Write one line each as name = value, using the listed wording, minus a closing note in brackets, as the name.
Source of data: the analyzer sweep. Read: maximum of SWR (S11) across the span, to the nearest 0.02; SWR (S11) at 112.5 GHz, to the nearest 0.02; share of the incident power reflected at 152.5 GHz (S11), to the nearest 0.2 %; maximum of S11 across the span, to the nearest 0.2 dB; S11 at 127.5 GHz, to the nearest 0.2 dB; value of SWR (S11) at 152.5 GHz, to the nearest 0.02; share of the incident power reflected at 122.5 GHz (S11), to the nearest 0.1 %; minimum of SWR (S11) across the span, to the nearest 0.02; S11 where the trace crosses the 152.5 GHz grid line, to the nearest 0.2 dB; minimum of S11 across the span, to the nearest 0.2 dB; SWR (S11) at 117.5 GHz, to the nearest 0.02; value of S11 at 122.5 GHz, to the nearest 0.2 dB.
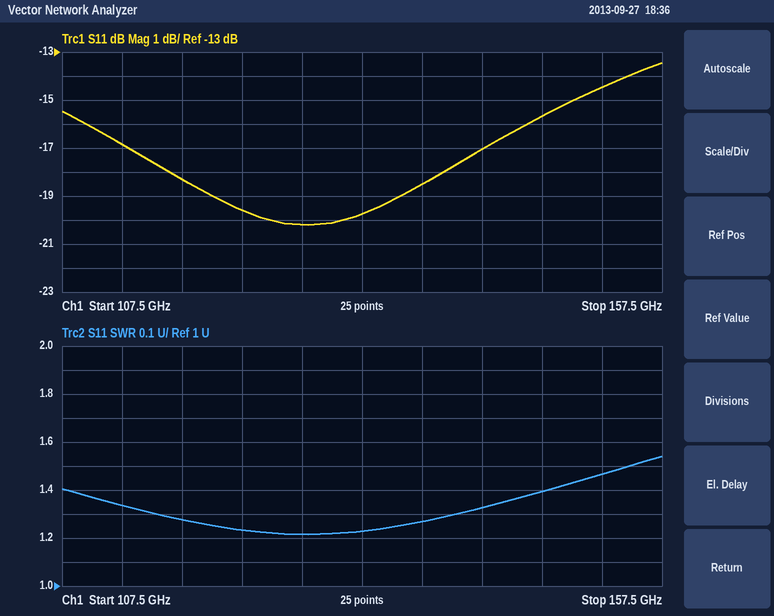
maximum of SWR (S11) across the span, to the nearest 0.02 = 1.54
SWR (S11) at 112.5 GHz, to the nearest 0.02 = 1.34
share of the incident power reflected at 152.5 GHz (S11), to the nearest 0.2 % = 3.6 %
maximum of S11 across the span, to the nearest 0.2 dB = -13.4 dB
S11 at 127.5 GHz, to the nearest 0.2 dB = -20.2 dB
value of SWR (S11) at 152.5 GHz, to the nearest 0.02 = 1.46
share of the incident power reflected at 122.5 GHz (S11), to the nearest 0.1 % = 1.1 %
minimum of SWR (S11) across the span, to the nearest 0.02 = 1.22
S11 where the trace crosses the 152.5 GHz grid line, to the nearest 0.2 dB = -14.4 dB
minimum of S11 across the span, to the nearest 0.2 dB = -20.2 dB
SWR (S11) at 117.5 GHz, to the nearest 0.02 = 1.28
value of S11 at 122.5 GHz, to the nearest 0.2 dB = -19.6 dB
